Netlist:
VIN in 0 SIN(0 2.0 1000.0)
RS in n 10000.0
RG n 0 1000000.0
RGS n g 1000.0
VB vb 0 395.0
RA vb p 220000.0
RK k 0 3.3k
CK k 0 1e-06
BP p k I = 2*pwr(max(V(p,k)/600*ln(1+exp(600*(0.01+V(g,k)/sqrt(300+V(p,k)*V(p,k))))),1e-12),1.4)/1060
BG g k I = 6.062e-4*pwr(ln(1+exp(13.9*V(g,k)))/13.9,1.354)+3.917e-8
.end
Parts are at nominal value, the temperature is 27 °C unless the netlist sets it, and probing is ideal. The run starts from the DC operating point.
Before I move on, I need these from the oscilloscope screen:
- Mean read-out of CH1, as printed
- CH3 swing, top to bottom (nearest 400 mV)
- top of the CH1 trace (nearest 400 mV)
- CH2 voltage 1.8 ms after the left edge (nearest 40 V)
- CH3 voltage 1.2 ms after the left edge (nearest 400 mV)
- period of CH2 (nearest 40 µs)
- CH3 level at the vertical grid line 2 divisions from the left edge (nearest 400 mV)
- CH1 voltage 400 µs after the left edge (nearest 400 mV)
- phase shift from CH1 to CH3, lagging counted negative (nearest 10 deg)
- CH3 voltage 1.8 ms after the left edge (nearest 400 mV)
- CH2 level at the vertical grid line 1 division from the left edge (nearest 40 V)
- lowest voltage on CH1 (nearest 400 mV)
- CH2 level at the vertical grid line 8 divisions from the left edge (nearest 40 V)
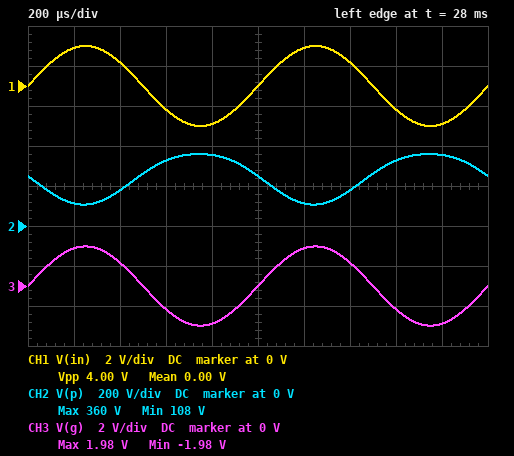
0.00 V
4.0 V
2.0 V
360 V
2.0 V
1.00 ms
1.2 V
1.2 V
0 deg
-2.0 V
120 V
-2.0 V
320 V
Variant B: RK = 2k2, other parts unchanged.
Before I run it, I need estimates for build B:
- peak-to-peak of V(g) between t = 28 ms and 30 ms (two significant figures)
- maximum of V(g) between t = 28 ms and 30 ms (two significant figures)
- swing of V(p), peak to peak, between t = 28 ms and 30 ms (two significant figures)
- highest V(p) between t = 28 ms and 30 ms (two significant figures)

3.8 V
1.8 V
260 V
340 V
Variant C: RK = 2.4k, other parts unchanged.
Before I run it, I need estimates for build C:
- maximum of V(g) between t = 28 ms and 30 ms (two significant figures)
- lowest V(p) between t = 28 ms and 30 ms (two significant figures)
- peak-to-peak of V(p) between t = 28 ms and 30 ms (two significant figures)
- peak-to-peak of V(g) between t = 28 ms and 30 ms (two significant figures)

1.9 V
85 V
260 V
3.9 V
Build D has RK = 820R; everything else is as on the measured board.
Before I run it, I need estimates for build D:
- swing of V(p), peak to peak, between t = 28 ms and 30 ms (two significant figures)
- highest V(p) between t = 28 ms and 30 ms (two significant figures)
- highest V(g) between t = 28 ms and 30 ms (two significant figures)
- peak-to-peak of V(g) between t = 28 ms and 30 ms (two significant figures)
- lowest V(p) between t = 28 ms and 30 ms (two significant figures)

230 V
290 V
1.1 V
3.1 V
65 V
